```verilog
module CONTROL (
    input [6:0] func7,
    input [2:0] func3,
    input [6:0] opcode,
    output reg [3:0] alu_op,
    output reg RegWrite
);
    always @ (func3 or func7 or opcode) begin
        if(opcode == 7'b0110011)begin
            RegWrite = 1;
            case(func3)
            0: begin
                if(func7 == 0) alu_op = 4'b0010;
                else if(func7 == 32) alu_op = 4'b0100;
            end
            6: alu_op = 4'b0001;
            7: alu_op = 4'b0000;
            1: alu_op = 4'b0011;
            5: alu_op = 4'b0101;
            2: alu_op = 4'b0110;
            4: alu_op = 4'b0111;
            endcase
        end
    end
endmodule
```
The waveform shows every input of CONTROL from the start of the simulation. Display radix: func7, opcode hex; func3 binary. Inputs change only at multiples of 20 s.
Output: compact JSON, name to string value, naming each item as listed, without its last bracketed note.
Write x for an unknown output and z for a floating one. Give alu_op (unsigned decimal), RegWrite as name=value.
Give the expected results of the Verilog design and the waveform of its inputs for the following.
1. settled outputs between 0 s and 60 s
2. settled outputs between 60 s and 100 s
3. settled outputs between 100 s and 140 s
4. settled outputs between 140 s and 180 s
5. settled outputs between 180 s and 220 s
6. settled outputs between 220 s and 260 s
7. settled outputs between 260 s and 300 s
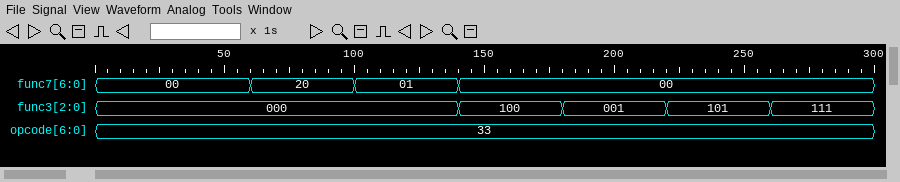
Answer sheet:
{"settled outputs between 0 s and 60 s": "alu_op=2, RegWrite=1", "settled outputs between 60 s and 100 s": "alu_op=4, RegWrite=1", "settled outputs between 100 s and 140 s": "alu_op=4, RegWrite=1", "settled outputs between 140 s and 180 s": "alu_op=7, RegWrite=1", "settled outputs between 180 s and 220 s": "alu_op=3, RegWrite=1", "settled outputs between 220 s and 260 s": "alu_op=5, RegWrite=1", "settled outputs between 260 s and 300 s": "alu_op=0, RegWrite=1"}
